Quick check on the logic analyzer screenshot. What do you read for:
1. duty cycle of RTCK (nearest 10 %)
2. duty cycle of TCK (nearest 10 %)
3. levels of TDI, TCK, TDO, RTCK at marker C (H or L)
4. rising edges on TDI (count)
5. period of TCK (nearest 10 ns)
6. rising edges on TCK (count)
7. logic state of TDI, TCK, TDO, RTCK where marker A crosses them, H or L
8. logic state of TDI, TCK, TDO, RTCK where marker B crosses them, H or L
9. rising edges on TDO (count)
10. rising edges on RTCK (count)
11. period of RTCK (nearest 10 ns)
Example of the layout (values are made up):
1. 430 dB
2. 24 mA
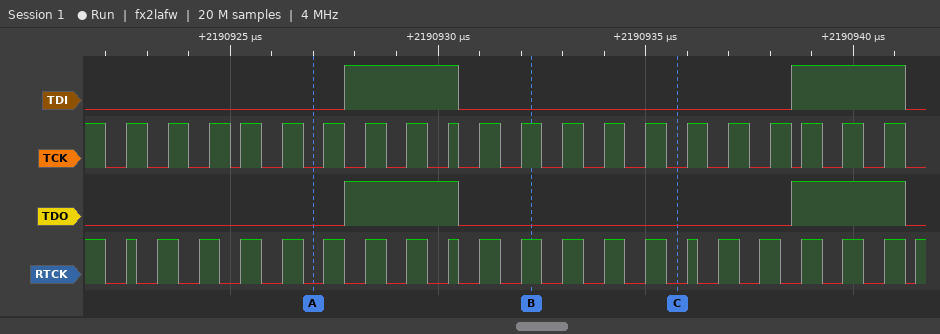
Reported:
1. 50 %
2. 50 %
3. TDI=L, TCK=L, TDO=L, RTCK=L
4. 2
5. 960 ns
6. 20
7. TDI=L, TCK=L, TDO=L, RTCK=L
8. TDI=L, TCK=H, TDO=L, RTCK=H
9. 2
10. 21
11. 950 ns
